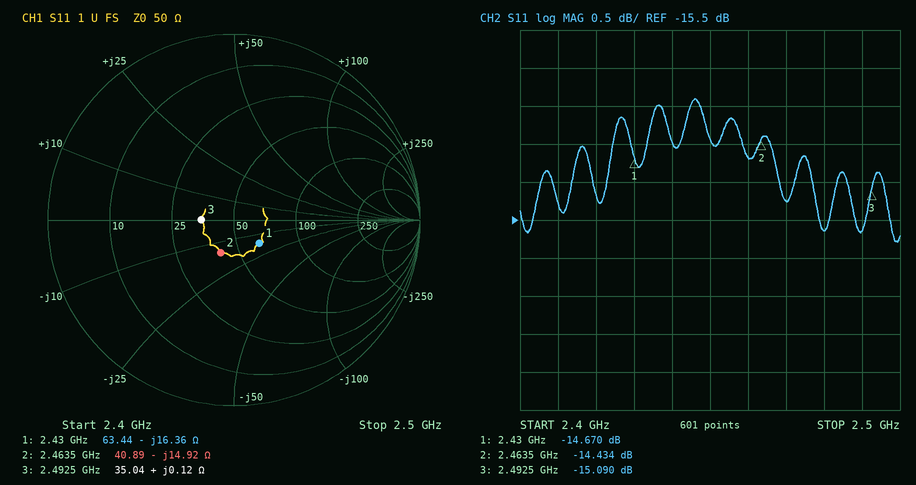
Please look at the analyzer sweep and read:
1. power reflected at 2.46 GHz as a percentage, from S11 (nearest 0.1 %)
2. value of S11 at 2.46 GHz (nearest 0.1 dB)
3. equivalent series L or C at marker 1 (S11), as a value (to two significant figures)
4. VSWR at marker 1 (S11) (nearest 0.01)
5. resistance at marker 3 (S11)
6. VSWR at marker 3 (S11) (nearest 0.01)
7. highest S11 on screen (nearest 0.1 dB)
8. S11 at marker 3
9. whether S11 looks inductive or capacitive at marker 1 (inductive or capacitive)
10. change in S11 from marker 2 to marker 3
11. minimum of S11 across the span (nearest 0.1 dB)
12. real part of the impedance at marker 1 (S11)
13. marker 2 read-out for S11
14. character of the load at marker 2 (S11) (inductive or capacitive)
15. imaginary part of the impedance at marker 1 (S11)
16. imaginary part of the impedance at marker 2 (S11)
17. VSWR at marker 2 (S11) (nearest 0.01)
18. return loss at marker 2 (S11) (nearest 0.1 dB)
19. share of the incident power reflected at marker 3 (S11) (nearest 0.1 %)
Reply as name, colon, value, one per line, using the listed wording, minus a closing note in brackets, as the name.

power reflected at 2.46 GHz as a percentage, from S11: 3.4 %
value of S11 at 2.46 GHz: -14.7 dB
equivalent series L or C at marker 1 (S11), as a value: 4.0 pF
VSWR at marker 1 (S11): 1.45
resistance at marker 3: 35.04 Ω
VSWR at marker 3 (S11): 1.43
highest S11 on screen: -13.9 dB
S11 at marker 3: -15.090 dB
whether S11 looks inductive or capacitive at marker 1: capacitive
change in S11 from marker 2 to marker 3: -0.656 dB
minimum of S11 across the span: -15.8 dB
real part of the impedance at marker 1: 63.44 Ω
marker 2 read-out for S11: -14.434 dB
character of the load at marker 2 (S11): capacitive
imaginary part of the impedance at marker 1: -16.36 Ω
imaginary part of the impedance at marker 2: -14.92 Ω
VSWR at marker 2 (S11): 1.47
return loss at marker 2 (S11): 14.4 dB
share of the incident power reflected at marker 3 (S11): 3.1 %
